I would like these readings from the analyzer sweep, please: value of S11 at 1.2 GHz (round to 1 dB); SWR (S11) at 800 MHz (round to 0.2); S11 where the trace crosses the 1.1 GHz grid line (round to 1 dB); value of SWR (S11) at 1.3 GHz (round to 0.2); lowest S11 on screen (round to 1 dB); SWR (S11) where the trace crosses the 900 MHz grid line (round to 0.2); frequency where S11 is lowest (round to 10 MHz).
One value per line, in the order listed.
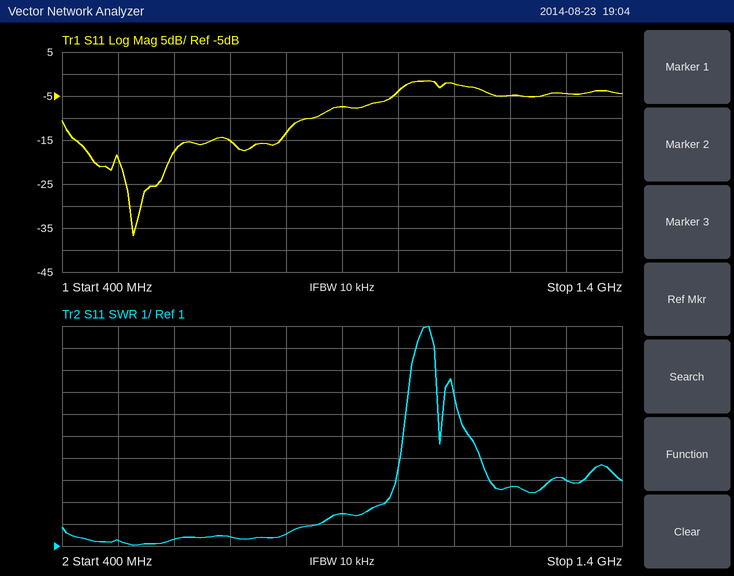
-5 dB
1.6
-2 dB
4.0
-37 dB
2.4
530 MHz
